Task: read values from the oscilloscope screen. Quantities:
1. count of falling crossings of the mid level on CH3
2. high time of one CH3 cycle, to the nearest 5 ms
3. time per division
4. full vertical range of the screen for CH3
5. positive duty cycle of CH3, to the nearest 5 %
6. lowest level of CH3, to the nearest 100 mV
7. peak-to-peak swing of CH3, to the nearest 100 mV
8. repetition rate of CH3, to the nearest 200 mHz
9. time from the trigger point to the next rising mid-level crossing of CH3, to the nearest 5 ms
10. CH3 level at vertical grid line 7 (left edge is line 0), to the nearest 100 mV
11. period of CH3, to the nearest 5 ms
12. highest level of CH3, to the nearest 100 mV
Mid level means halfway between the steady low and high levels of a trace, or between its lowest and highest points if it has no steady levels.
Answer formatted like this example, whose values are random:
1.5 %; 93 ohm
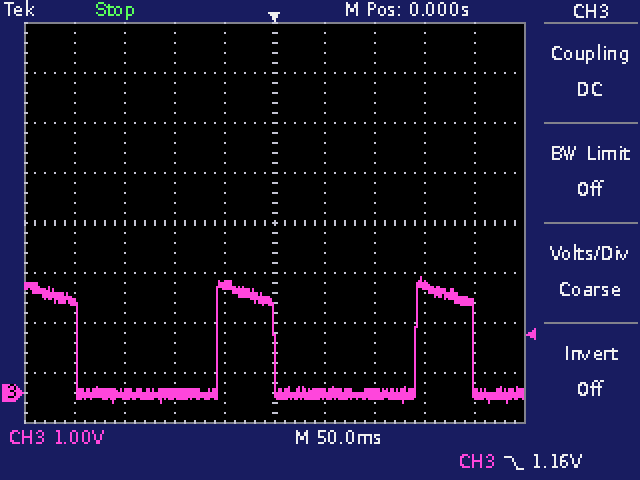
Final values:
3; 55 ms; 50 ms; 8 V; 30 %; -200 mV; 2.5 V; 5.0 Hz; 140 ms; 0.0 V; 200 ms; 2.3 V
